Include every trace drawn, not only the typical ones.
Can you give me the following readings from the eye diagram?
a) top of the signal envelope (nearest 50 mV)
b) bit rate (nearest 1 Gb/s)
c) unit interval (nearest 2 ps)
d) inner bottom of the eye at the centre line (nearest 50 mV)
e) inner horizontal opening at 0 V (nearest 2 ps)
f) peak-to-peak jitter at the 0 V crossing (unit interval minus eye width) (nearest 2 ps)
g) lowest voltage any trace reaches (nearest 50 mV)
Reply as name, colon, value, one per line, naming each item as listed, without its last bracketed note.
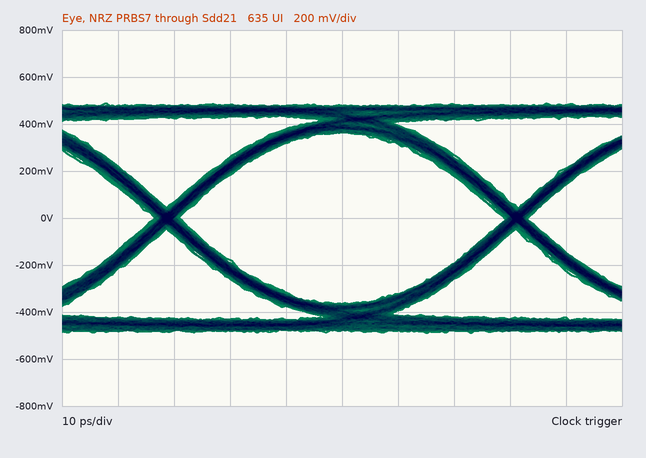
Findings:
top of the signal envelope: 500 mV
bit rate: 16 Gb/s
unit interval: 62 ps
inner bottom of the eye at the centre line: -350 mV
inner horizontal opening at 0 V: 58 ps
peak-to-peak jitter at the 0 V crossing (unit interval minus eye width): 4 ps
lowest voltage any trace reaches: -500 mV
